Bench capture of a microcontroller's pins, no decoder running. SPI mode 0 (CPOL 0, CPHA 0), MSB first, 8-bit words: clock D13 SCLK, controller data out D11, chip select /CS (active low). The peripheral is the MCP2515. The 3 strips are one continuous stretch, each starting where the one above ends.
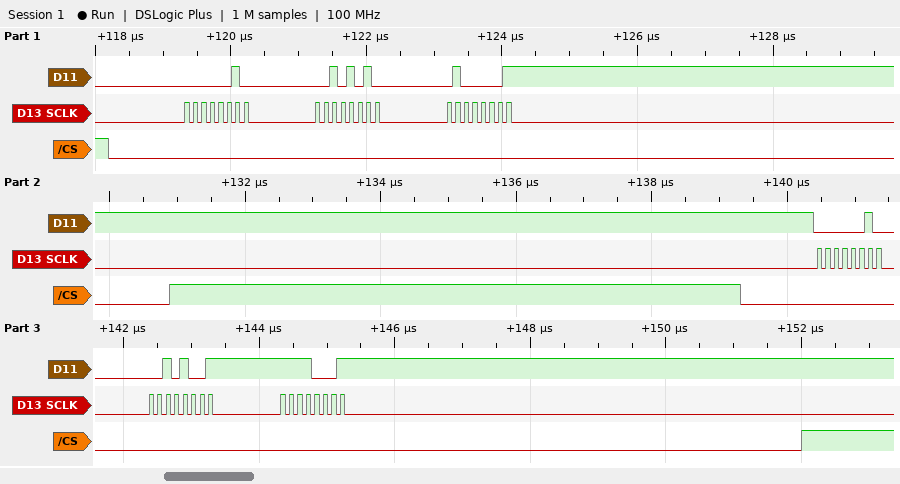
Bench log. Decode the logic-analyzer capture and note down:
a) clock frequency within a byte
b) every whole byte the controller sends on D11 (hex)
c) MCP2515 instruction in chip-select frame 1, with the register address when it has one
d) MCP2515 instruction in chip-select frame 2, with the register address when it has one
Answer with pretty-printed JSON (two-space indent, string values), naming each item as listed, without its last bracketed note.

{
  "clock frequency within a byte": "8 MHz",
  "every whole byte the controller sends on D11": "02 2A 41 02 29 F1",
  "MCP2515 instruction in chip-select frame 1, with the register address when it has one": "WRITE 0x2A",
  "MCP2515 instruction in chip-select frame 2, with the register address when it has one": "WRITE 0x29"
}
